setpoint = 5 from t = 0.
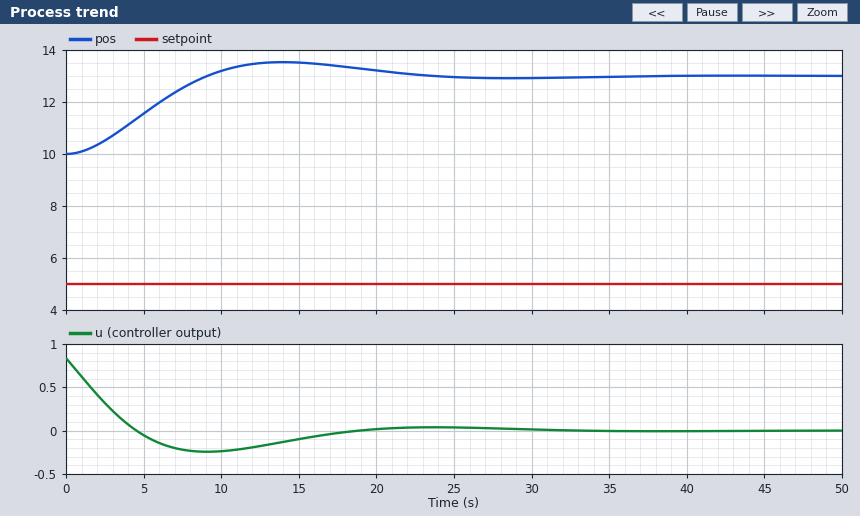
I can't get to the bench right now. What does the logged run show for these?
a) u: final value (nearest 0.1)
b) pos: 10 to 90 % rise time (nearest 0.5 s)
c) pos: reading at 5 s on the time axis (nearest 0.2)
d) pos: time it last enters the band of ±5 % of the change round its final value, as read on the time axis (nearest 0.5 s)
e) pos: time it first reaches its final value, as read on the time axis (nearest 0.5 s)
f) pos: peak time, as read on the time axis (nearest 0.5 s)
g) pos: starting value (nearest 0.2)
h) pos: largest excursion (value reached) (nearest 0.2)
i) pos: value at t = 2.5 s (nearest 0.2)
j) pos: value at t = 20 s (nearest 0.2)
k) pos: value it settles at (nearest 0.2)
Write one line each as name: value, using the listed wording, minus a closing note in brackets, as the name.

u: final value: 0.0
pos: 10 to 90 % rise time: 6.0 s
pos: reading at 5 s on the time axis: 11.6
pos: time it last enters the band of ±5 % of the change round its final value, as read on the time axis: 21.0 s
pos: time it first reaches its final value, as read on the time axis: 9.0 s
pos: peak time, as read on the time axis: 14.0 s
pos: starting value: 10.0
pos: largest excursion (value reached): 13.6
pos: value at t = 2.5 s: 10.6
pos: value at t = 20 s: 13.2
pos: value it settles at: 13.0
